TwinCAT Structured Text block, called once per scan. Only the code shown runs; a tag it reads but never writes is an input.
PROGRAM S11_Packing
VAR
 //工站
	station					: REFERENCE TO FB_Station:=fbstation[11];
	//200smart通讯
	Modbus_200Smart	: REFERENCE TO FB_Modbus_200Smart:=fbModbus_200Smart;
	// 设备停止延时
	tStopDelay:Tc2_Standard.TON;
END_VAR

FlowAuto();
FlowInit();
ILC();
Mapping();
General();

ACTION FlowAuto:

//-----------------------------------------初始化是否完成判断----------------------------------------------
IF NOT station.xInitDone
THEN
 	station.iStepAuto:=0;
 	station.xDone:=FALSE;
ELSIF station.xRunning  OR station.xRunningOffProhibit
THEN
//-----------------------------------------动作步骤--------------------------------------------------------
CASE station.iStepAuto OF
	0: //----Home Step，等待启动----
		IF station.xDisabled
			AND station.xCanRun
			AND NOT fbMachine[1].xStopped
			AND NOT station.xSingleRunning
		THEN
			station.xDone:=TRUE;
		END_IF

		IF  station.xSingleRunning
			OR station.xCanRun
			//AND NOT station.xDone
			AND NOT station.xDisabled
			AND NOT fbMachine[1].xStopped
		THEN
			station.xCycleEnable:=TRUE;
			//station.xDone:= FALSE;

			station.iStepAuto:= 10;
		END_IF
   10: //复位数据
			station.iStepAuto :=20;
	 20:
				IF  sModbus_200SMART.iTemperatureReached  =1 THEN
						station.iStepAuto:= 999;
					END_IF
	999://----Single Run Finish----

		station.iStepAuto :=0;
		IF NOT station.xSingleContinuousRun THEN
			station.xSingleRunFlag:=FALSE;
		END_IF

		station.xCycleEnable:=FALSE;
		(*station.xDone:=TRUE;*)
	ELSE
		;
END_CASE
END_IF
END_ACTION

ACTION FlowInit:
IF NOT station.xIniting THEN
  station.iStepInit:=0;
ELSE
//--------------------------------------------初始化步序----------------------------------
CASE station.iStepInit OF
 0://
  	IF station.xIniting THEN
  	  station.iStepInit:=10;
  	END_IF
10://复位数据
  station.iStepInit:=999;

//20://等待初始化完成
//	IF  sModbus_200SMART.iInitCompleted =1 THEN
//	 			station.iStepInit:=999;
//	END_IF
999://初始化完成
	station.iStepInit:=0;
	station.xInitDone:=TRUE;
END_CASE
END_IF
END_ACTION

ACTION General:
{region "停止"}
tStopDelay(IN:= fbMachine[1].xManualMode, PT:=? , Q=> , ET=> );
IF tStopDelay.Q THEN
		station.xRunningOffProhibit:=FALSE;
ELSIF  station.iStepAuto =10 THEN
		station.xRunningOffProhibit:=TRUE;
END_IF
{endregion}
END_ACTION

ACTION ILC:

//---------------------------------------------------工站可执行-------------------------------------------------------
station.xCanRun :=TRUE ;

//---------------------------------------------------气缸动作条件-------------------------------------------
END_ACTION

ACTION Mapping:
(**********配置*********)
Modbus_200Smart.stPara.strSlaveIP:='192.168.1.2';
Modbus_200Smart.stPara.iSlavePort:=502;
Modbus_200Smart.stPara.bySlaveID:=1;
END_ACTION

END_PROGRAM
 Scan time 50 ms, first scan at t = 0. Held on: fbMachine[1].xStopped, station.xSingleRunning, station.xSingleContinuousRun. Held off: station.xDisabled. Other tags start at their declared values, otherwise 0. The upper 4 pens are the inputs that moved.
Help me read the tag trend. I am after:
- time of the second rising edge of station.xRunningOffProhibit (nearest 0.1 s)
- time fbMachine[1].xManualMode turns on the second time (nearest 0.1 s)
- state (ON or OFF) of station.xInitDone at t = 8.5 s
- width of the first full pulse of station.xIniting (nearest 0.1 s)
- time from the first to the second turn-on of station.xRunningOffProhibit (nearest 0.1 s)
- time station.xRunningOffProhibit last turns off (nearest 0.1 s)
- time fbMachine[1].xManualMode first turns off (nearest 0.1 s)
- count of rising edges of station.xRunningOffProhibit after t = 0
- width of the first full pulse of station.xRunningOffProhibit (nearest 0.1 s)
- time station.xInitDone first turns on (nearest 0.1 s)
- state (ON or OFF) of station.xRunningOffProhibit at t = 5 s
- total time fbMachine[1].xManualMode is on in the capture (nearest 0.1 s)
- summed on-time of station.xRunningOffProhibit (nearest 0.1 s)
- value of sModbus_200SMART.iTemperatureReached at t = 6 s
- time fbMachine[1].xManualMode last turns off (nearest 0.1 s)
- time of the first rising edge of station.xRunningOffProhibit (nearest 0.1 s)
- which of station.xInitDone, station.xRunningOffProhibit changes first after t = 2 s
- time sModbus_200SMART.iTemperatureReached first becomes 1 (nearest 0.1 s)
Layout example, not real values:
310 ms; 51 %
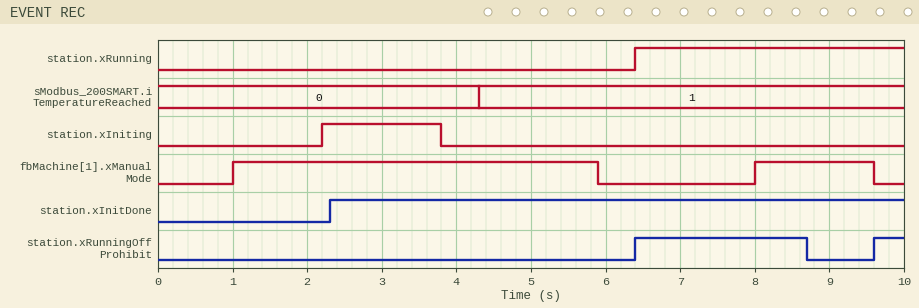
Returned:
9.6 s; 8.0 s; ON; 1.6 s; 3.2 s; 8.7 s; 5.9 s; 2; 2.3 s; 2.3 s; OFF; 6.5 s; 2.7 s; 1; 9.6 s; 6.4 s; station.xInitDone; 4.3 s
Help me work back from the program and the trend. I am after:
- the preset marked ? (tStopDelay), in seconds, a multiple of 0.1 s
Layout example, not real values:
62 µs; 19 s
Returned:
0.7 s
